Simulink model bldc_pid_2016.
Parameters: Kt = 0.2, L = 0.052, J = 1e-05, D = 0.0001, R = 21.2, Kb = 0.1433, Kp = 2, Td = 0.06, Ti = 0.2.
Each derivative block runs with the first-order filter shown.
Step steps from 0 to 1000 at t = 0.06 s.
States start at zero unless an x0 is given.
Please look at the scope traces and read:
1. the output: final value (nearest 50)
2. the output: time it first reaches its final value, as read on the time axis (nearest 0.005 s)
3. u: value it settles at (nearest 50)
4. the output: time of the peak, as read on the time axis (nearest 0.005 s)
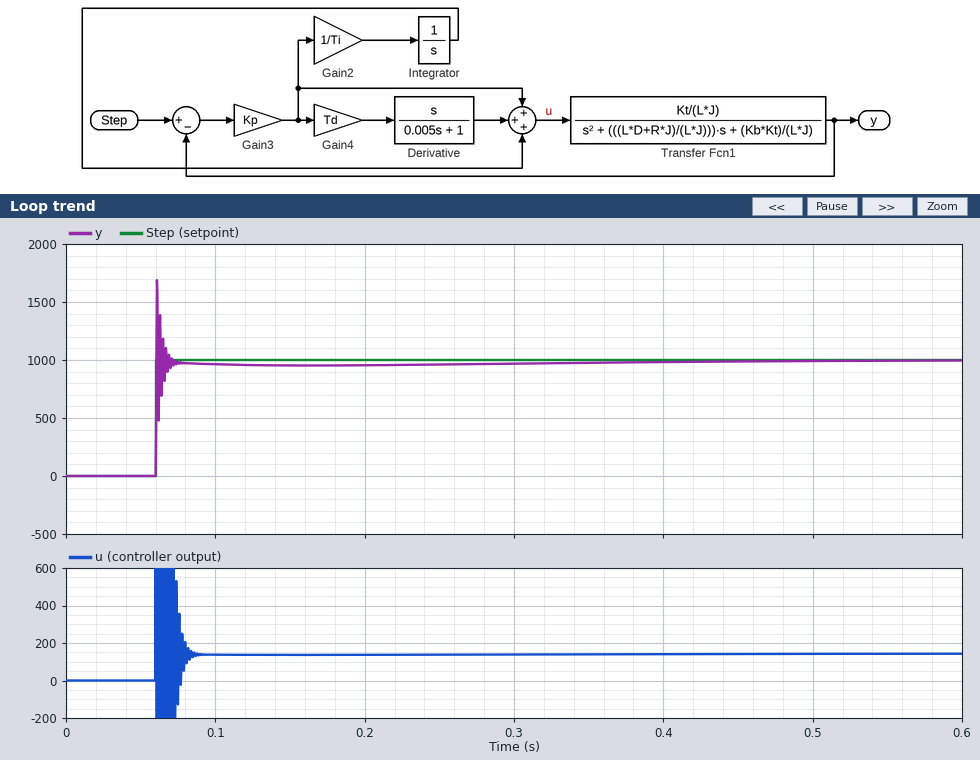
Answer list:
1000
0.060 s
150
0.060 s
